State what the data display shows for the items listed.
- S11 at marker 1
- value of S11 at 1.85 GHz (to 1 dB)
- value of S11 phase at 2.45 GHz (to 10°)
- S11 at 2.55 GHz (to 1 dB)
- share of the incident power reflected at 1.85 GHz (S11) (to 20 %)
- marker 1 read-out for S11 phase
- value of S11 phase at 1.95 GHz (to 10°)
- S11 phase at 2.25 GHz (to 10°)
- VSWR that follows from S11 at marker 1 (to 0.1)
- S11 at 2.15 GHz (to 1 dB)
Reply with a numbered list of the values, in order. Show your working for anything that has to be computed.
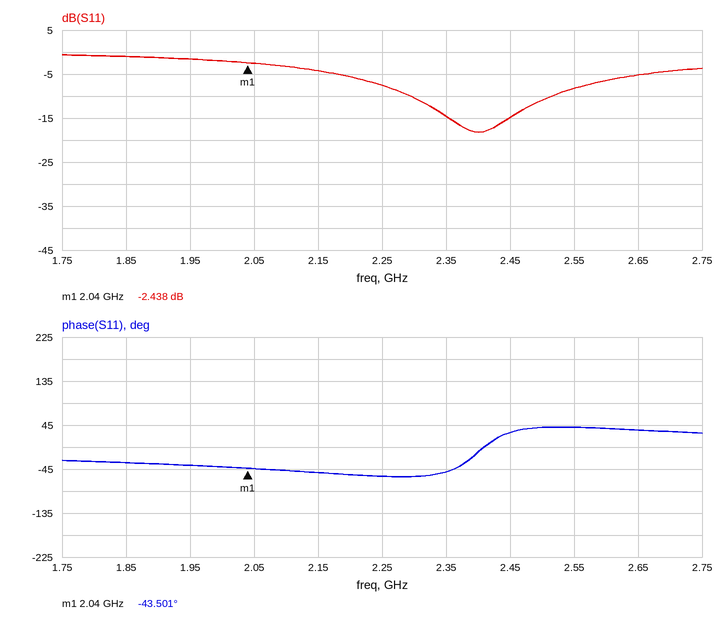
1. -2.438 dB
2. -1 dB
3. 30°
4. -8 dB
5. 10^(-1/10) ≈ 79.4 %, so 80 % to the nearest 20 %
6. -43.501°
7. -40°
8. -60°
9. (1 + 0.7553)/(1 − 0.7553) ≈ 7.2
10. -4 dB
